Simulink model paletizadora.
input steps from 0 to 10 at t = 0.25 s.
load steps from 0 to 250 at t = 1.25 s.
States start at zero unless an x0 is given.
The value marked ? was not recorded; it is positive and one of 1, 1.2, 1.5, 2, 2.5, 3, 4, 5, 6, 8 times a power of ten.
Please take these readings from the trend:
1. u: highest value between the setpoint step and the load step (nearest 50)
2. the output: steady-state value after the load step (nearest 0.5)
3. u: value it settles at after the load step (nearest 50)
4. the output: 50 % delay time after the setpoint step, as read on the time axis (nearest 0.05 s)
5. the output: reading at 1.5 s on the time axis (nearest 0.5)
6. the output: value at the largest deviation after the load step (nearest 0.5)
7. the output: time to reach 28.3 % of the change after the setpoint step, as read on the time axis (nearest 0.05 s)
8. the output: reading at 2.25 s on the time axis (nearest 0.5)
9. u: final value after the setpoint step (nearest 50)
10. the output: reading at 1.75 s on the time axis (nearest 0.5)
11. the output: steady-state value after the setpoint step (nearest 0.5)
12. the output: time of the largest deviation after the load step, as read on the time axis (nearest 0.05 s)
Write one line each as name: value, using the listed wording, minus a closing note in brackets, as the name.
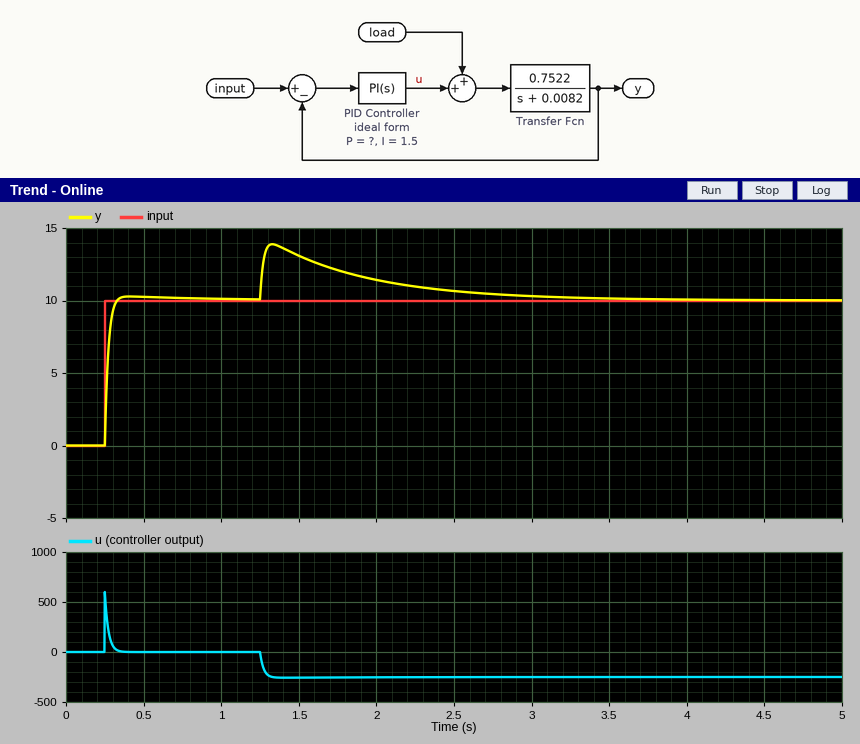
u: highest value between the setpoint step and the load step: 600
the output: steady-state value after the load step: 10.0
u: value it settles at after the load step: -250
the output: 50 % delay time after the setpoint step, as read on the time axis: 0.25 s
the output: reading at 1.5 s on the time axis: 13.0
the output: value at the largest deviation after the load step: 14.0
the output: time to reach 28.3 % of the change after the setpoint step, as read on the time axis: 0.25 s
the output: reading at 2.25 s on the time axis: 11.0
u: final value after the setpoint step: 0
the output: reading at 1.75 s on the time axis: 12.0
the output: steady-state value after the setpoint step: 10.0
the output: time of the largest deviation after the load step, as read on the time axis: 1.35 s
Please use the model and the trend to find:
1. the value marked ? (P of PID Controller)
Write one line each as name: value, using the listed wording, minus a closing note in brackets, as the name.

the value marked ?: 60
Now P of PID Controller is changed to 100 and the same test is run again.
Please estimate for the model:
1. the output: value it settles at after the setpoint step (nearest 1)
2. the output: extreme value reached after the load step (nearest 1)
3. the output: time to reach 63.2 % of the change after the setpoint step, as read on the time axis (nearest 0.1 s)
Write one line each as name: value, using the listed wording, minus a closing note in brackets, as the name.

the output: value it settles at after the setpoint step: 10
the output: extreme value reached after the load step: 12
the output: time to reach 63.2 % of the change after the setpoint step, as read on the time axis: 0.3 s
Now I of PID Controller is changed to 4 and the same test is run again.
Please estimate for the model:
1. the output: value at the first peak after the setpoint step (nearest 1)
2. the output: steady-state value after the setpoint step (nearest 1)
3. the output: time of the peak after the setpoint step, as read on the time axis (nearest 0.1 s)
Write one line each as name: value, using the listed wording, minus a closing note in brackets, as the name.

the output: value at the first peak after the setpoint step: 11
the output: steady-state value after the setpoint step: 10
the output: time of the peak after the setpoint step, as read on the time axis: 0.4 s
